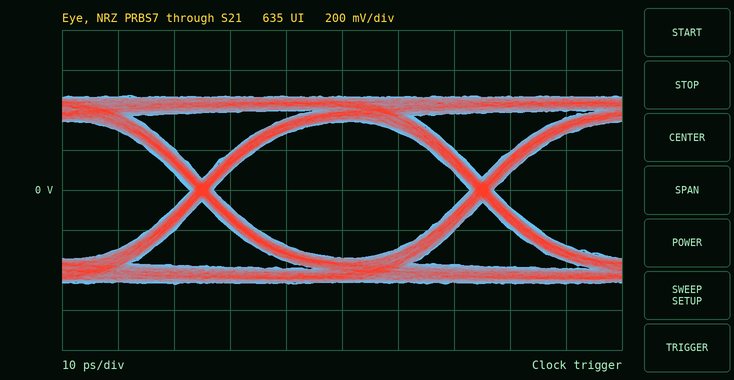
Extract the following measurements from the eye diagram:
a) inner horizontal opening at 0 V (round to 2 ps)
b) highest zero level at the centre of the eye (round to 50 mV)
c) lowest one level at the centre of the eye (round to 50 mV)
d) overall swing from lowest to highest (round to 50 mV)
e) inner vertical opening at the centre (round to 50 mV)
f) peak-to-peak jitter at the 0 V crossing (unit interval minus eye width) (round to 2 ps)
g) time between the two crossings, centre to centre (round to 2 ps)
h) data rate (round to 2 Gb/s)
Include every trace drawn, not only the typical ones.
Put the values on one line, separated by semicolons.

46 ps; -350 mV; 350 mV; 950 mV; 700 mV; 4 ps; 50 ps; 20 Gb/s
